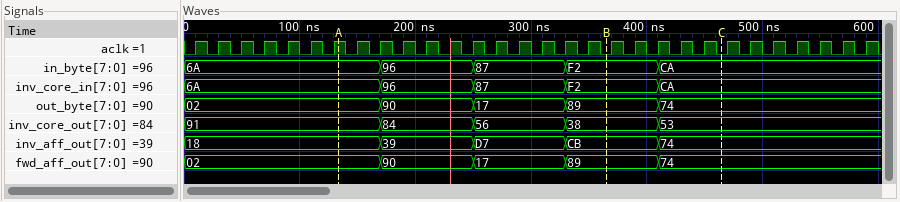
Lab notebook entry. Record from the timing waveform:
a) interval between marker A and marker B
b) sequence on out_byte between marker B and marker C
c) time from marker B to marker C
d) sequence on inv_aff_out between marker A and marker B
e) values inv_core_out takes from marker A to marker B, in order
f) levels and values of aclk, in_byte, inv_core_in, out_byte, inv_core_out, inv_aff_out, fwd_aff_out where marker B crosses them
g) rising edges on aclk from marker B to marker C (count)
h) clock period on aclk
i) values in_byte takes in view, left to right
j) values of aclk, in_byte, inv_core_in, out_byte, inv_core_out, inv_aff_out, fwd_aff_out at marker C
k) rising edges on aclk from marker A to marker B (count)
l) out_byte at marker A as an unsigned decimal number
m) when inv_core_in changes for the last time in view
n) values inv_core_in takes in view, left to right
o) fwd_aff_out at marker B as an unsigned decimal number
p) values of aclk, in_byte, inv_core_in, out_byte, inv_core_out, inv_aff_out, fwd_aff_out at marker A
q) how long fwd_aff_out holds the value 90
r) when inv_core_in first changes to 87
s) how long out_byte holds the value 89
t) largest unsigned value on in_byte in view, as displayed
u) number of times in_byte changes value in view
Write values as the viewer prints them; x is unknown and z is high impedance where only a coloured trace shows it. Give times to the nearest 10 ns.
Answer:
230 ns
89, 74
100 ns
18, 39, D7, CB
91, 84, 56, 38
aclk=0, in_byte=F2, inv_core_in=F2, out_byte=89, inv_core_out=38, inv_aff_out=CB, fwd_aff_out=89
5
20 ns
6A, 96, 87, F2, CA
aclk=0, in_byte=CA, inv_core_in=CA, out_byte=74, inv_core_out=53, inv_aff_out=74, fwd_aff_out=74
11
2
410 ns
6A, 96, 87, F2, CA
137
aclk=1, in_byte=6A, inv_core_in=6A, out_byte=02, inv_core_out=91, inv_aff_out=18, fwd_aff_out=02
80 ns
250 ns
80 ns
F2
4
